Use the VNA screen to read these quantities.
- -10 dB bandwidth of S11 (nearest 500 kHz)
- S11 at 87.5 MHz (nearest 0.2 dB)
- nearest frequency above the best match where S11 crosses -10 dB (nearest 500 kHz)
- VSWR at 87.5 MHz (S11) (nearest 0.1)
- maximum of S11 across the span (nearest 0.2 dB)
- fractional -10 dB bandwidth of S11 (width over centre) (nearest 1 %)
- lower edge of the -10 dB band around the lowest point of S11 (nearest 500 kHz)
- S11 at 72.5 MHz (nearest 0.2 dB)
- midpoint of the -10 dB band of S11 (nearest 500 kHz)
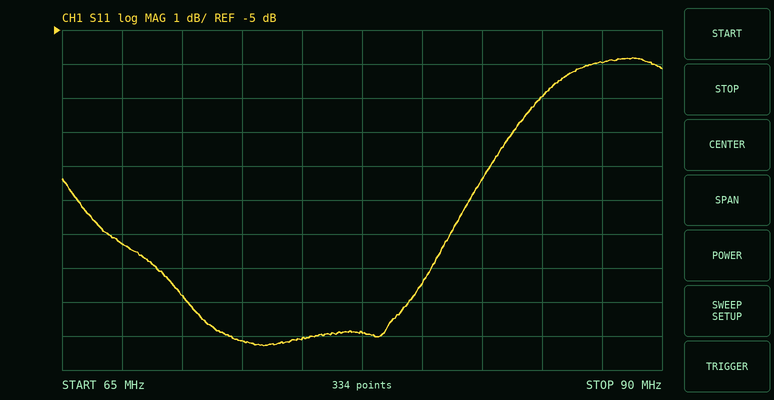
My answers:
16.5 MHz
-6.0 dB
82.0 MHz
3.0
-5.8 dB
22 %
65.5 MHz
-14.2 dB
74.0 MHz
